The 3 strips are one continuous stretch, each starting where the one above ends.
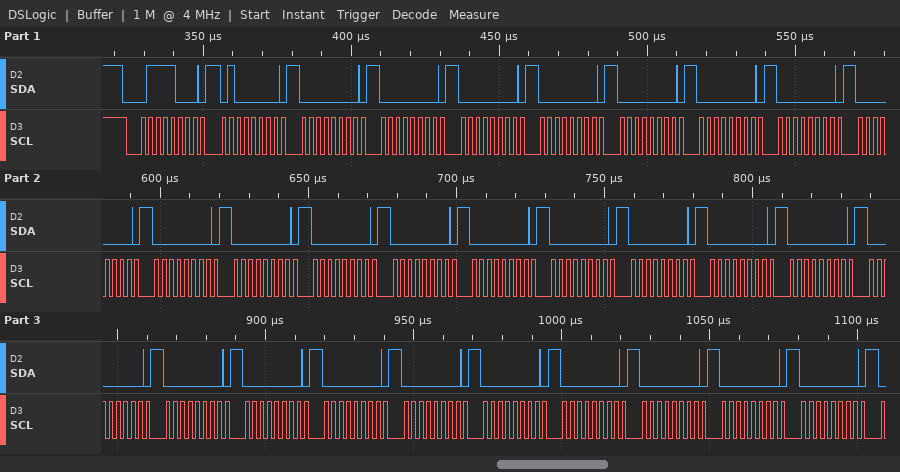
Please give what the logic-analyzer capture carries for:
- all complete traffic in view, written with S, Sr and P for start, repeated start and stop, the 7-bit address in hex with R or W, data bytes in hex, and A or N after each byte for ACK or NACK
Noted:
S 3CW A 40 A 00 A 00 A 00 A 00 A 00 A 00 A 00 A 00 A 00 A 00 A 00 A 00 A 00 A 00 A 00 A 00 A 00 A 00 A 00 A 00 A 00 A 00 A 00 A 00 A 00 A 00 A 00 A
